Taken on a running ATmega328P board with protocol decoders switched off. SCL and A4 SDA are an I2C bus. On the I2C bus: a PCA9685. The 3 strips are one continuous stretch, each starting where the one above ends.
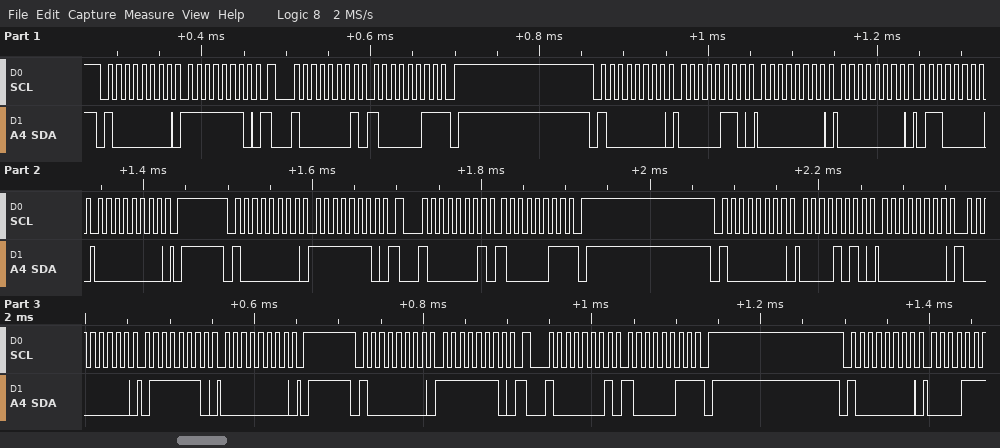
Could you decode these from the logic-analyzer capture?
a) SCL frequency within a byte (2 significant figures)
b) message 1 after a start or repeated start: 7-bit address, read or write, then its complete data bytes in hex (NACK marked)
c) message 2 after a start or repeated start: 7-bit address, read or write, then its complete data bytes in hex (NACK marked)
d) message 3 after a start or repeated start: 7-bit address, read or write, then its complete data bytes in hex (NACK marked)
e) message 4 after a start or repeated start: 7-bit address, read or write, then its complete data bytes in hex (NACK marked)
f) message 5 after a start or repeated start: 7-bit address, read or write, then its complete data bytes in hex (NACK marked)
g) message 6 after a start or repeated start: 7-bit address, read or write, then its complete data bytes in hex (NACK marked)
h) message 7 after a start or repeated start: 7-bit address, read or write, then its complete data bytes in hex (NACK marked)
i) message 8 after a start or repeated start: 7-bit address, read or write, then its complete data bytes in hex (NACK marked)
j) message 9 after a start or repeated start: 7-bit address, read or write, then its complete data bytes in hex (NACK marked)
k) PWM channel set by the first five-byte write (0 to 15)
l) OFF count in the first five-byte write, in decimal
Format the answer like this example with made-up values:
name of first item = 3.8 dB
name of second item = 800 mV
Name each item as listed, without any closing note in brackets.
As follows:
SCL frequency within a byte = 100 kHz
message 1 after a start or repeated start: 7-bit address, read or write, then its complete data bytes in hex = 0x40 write: FE
message 2 after a start or repeated start: 7-bit address, read or write, then its complete data bytes in hex = 0x40 read: 83 NACK
message 3 after a start or repeated start: 7-bit address, read or write, then its complete data bytes in hex = 0x40 write: 06 00 00 60 00
message 4 after a start or repeated start: 7-bit address, read or write, then its complete data bytes in hex = 0x40 write: FE
message 5 after a start or repeated start: 7-bit address, read or write, then its complete data bytes in hex = 0x40 read: 83 NACK
message 6 after a start or repeated start: 7-bit address, read or write, then its complete data bytes in hex = 0x40 write: 0A 00 00 7E 00
message 7 after a start or repeated start: 7-bit address, read or write, then its complete data bytes in hex = 0x40 write: FE
message 8 after a start or repeated start: 7-bit address, read or write, then its complete data bytes in hex = 0x40 read: 83 NACK
message 9 after a start or repeated start: 7-bit address, read or write, then its complete data bytes in hex = 0x40 write
PWM channel set by the first five-byte write = 0
OFF count in the first five-byte write, in decimal = 96
